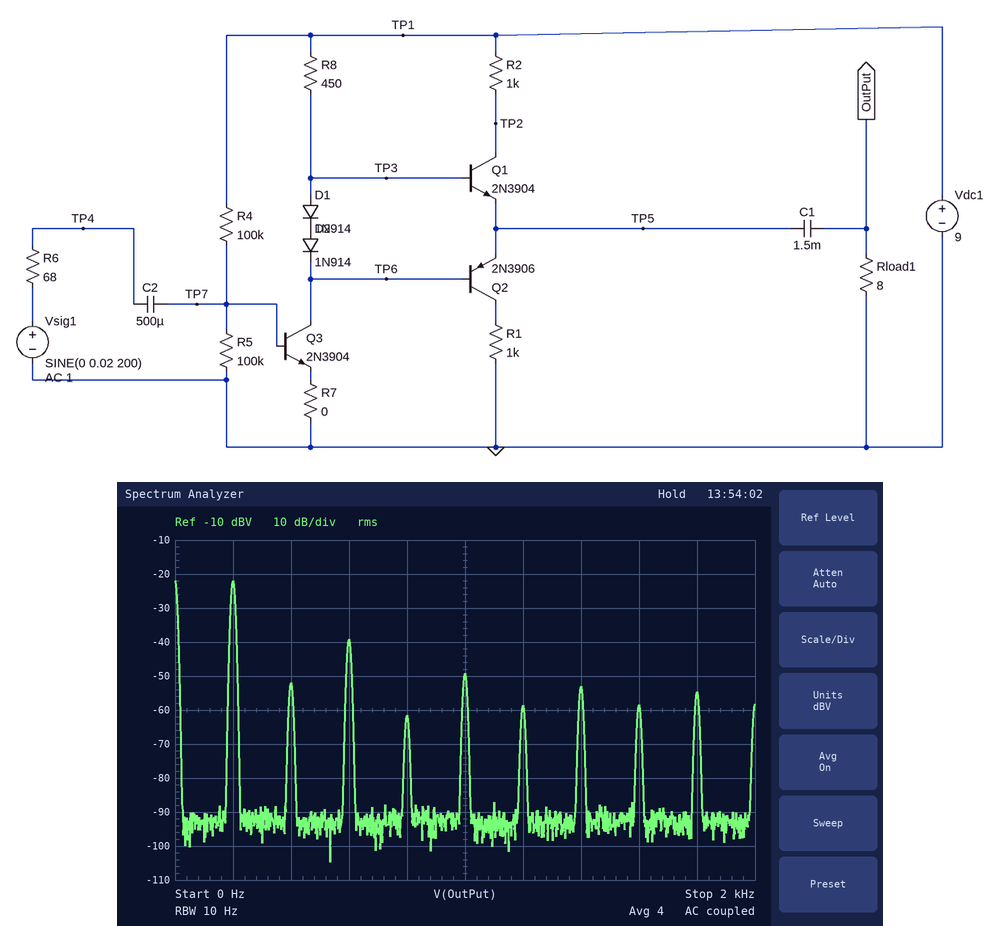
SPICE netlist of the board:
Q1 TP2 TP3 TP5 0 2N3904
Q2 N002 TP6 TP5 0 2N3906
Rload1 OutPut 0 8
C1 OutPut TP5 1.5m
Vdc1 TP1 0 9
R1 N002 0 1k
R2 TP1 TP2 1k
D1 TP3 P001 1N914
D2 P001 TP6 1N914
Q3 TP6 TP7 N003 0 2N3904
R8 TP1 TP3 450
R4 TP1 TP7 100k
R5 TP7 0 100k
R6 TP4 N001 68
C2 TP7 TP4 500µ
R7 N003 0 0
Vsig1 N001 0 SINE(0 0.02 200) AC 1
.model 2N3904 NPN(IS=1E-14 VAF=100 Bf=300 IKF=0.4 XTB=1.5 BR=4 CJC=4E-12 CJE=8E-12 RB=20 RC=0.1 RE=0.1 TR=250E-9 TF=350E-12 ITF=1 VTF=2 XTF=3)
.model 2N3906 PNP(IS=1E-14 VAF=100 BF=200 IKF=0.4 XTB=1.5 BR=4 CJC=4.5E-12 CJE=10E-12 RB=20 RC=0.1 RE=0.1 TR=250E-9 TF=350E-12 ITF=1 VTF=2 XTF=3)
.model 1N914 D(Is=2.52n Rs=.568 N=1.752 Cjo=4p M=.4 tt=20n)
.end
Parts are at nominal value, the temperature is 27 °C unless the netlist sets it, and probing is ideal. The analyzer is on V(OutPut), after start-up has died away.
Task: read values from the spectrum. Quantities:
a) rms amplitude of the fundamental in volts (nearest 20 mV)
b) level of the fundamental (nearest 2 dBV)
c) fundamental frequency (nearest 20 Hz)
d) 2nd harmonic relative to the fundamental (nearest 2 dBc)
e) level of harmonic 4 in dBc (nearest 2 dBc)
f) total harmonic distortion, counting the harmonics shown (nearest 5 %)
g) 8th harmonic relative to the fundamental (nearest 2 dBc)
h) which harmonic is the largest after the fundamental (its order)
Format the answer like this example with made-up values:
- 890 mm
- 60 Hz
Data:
- 80 mV
- -22 dBV
- 200 Hz
- -30 dBc
- -40 dBc
- 15 %
- -36 dBc
- 3
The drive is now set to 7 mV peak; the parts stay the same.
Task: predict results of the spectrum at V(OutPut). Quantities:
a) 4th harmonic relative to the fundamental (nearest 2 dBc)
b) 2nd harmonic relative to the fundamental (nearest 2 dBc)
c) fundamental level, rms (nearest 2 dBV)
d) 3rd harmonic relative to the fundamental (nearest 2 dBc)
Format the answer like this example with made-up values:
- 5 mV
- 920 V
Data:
- -20 dBc
- -14 dBc
- -28 dBV
- -18 dBc
